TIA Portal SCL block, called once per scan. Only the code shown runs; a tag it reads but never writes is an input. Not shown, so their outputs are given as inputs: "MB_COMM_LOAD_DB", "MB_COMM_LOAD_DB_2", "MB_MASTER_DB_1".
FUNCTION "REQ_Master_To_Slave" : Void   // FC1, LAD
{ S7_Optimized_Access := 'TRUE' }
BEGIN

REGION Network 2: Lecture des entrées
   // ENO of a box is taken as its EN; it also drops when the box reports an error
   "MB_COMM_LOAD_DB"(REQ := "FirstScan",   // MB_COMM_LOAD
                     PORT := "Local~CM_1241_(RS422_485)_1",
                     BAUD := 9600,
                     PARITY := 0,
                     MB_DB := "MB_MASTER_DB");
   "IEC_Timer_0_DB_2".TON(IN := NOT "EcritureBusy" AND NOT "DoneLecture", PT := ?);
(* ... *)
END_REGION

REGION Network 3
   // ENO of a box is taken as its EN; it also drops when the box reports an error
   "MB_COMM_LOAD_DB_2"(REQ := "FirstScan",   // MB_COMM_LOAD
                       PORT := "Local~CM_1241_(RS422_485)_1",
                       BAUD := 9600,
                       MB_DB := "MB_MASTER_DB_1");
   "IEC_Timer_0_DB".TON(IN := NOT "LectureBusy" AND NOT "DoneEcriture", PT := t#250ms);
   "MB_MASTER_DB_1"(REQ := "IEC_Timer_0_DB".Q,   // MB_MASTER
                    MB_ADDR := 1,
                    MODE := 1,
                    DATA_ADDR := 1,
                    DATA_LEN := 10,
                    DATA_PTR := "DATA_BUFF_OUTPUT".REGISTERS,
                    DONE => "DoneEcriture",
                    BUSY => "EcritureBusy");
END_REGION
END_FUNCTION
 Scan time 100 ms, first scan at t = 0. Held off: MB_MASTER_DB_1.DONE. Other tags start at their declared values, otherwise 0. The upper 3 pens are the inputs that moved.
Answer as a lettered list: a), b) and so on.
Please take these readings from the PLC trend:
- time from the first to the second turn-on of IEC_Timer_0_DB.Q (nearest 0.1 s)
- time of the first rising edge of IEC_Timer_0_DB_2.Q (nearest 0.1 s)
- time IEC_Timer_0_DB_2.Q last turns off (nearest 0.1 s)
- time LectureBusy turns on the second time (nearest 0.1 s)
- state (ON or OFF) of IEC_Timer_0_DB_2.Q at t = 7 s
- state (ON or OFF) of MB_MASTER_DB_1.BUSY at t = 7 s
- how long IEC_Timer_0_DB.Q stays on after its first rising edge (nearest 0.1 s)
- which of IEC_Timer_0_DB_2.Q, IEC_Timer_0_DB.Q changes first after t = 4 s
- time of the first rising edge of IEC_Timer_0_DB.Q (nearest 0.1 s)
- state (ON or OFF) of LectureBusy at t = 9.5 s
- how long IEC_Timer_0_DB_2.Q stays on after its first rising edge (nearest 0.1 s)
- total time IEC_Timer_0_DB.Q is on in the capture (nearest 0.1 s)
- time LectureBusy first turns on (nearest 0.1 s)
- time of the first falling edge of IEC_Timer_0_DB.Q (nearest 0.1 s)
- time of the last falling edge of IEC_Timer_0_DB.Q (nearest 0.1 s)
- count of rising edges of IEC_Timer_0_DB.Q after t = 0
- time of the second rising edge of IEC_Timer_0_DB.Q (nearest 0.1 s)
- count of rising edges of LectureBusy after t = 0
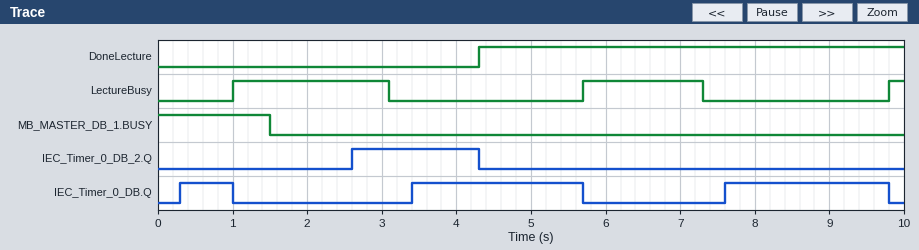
a) 3.1 s
b) 2.6 s
c) 4.3 s
d) 5.7 s
e) OFF
f) OFF
g) 0.7 s
h) IEC_Timer_0_DB_2.Q
i) 0.3 s
j) OFF
k) 1.7 s
l) 5.2 s
m) 1.0 s
n) 1.0 s
o) 9.8 s
p) 3
q) 3.4 s
r) 3
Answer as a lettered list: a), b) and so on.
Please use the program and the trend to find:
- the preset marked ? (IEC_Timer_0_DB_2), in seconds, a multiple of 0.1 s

a) 1.0 s
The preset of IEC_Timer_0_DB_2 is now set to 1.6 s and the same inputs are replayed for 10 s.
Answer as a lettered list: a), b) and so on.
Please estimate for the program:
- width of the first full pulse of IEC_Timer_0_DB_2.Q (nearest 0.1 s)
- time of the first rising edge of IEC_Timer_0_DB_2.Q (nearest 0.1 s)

a) 1.1 s
b) 3.2 s
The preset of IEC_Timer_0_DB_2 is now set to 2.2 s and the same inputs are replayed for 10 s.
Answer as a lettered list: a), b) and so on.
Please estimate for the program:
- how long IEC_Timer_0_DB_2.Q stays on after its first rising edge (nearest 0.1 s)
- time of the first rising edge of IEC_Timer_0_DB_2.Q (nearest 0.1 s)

a) 0.5 s
b) 3.8 s
